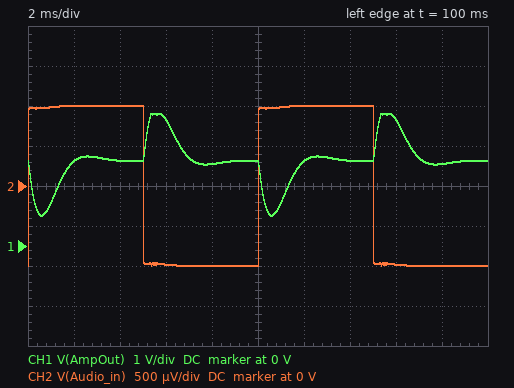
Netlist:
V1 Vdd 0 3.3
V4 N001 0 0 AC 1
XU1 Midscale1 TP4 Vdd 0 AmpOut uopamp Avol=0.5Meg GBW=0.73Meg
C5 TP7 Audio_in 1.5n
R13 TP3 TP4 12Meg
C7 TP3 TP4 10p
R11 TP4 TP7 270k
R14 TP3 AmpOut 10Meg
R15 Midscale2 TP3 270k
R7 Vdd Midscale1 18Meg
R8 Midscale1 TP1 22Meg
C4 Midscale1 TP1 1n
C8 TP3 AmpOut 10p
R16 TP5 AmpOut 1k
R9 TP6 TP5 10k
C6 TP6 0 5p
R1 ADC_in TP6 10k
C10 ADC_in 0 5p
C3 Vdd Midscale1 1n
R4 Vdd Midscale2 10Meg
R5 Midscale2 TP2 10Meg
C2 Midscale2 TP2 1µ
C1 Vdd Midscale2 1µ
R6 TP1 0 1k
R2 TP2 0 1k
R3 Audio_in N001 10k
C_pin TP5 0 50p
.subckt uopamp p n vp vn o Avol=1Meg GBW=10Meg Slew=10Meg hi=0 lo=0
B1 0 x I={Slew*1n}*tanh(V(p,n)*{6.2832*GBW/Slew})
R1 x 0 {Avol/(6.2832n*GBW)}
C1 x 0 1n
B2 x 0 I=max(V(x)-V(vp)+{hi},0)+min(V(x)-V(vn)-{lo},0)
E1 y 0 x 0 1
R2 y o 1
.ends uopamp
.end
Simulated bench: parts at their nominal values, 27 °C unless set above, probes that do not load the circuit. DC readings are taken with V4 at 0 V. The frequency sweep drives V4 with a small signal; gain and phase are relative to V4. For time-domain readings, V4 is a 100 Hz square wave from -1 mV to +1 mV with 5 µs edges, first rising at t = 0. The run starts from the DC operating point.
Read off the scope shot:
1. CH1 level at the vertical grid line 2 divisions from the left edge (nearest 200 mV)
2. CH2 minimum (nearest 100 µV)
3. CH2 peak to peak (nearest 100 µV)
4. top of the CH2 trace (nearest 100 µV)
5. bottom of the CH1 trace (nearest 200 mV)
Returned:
2.2 V
-1.0 mV
2.0 mV
1.0 mV
800 mV
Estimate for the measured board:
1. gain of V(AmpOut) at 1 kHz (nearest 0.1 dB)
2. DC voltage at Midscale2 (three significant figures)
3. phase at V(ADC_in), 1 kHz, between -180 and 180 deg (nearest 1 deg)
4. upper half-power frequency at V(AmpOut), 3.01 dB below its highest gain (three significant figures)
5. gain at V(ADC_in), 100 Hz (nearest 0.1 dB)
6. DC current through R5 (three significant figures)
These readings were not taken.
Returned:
53.2 dB
1.81 V
107 deg
580 Hz
53.0 dB
181 nA
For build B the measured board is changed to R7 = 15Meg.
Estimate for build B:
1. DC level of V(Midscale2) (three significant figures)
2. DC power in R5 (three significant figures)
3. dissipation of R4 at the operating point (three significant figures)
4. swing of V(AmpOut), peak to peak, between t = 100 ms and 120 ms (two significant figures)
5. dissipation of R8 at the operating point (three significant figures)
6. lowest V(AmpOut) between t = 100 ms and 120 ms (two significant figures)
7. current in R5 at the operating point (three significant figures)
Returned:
1.95 V
379 nW
183 nW
2.1 V
175 nW
1.2 V
195 nA
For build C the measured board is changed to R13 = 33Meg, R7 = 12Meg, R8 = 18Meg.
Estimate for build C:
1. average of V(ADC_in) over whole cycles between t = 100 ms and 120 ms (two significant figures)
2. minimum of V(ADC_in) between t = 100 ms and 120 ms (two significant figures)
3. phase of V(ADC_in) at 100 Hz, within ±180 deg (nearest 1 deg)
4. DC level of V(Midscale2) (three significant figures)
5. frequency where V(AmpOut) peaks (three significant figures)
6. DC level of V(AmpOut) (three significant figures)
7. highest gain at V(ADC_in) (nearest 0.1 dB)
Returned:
2.6 V
190 mV
-125 deg
1.96 V
204 Hz
2.61 V
67.1 dB
